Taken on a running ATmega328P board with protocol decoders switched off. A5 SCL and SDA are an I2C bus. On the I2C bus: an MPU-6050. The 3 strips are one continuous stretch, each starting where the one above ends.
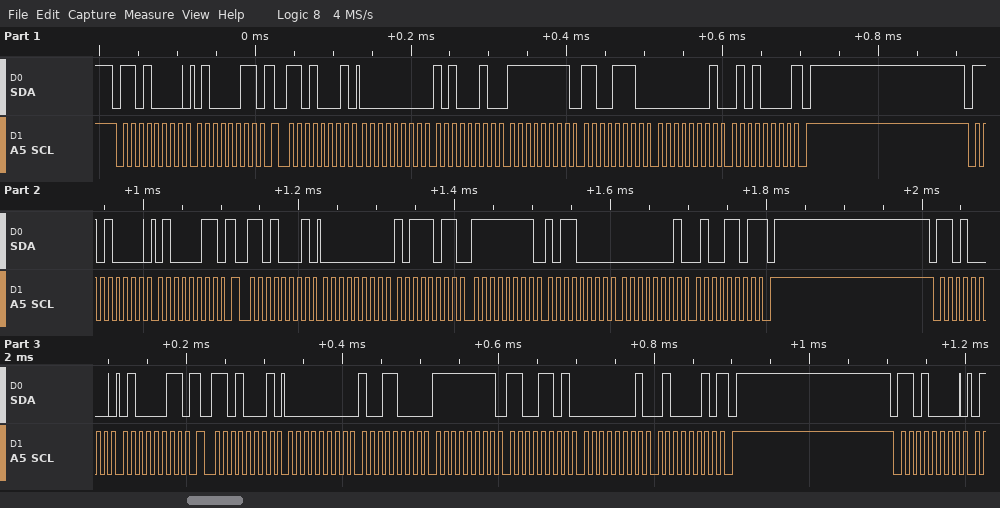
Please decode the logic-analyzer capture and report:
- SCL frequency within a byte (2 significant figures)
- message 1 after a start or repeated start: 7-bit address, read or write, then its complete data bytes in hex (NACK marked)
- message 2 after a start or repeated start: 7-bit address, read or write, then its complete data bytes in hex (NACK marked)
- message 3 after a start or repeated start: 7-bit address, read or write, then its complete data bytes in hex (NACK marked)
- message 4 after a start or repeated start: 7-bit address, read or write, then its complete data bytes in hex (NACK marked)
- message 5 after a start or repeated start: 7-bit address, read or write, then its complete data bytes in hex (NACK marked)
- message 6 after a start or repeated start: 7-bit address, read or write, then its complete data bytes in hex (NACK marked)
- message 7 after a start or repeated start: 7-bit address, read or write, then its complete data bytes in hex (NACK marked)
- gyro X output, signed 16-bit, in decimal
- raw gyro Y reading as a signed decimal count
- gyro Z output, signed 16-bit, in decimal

100 kHz
0x68 write: 43
0x68 read: 00 A2 FF CE 01 50 NACK
0x68 write: 43
0x68 read: 00 BB FF B0 01 4D NACK
0x68 write: 43
0x68 read: 00 98 FF CD 01 42 NACK
0x68 write
162
-50
336
